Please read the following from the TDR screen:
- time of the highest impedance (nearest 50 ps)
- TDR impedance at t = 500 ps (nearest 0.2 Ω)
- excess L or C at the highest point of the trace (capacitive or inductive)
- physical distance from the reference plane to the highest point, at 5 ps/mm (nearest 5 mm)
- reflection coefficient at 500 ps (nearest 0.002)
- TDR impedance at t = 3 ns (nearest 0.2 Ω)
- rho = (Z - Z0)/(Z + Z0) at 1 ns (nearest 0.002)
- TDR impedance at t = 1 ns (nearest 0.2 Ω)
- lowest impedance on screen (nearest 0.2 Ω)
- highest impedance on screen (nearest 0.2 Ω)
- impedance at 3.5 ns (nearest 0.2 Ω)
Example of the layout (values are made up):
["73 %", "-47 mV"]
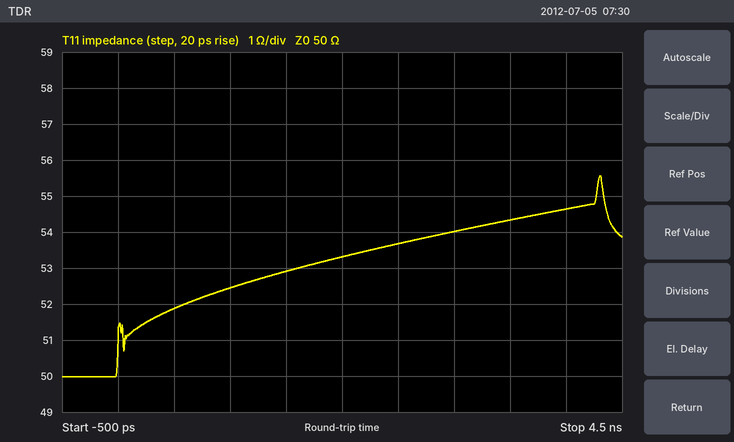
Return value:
["4.30 ns", "51.8 Ω", "inductive", "430 mm", "+0.018", "54.0 Ω", "+0.024", "52.4 Ω", "50.0 Ω", "55.6 Ω", "54.4 Ω"]
